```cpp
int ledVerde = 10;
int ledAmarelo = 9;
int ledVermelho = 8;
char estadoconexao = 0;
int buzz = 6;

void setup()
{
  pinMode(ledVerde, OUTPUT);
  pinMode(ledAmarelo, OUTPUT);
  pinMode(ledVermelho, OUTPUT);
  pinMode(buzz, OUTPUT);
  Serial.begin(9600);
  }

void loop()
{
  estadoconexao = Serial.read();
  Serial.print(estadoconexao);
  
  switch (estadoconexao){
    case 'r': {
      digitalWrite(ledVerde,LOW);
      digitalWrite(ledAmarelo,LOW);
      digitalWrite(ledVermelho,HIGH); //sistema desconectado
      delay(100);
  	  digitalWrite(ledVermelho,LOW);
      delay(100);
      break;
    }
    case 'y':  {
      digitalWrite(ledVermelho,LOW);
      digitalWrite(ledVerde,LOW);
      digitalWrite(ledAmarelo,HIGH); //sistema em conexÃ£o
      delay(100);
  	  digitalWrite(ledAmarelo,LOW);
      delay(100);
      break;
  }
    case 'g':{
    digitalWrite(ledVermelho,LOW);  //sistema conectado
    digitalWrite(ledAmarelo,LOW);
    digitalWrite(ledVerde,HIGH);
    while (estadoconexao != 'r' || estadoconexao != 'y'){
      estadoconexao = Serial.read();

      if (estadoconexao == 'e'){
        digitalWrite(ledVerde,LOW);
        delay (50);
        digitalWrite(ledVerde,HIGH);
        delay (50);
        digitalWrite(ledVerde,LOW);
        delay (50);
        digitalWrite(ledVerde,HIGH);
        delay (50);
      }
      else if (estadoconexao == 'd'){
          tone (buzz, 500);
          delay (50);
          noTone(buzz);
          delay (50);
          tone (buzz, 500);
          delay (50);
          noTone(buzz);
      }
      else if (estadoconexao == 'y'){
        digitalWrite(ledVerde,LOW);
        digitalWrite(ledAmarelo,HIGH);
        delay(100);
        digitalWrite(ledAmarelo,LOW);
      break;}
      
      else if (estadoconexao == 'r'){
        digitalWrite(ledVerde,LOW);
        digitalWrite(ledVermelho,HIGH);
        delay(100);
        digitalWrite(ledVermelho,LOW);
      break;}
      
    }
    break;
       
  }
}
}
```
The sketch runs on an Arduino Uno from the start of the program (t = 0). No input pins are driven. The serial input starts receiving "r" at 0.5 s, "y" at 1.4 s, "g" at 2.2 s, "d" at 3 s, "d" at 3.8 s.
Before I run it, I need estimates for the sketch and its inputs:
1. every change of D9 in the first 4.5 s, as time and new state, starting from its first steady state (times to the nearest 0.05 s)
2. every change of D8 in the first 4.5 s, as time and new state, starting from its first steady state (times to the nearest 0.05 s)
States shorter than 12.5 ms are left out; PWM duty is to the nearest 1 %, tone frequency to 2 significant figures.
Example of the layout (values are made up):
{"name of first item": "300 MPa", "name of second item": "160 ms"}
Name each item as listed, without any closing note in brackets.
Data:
{"every change of D9 in the first 4.5 s, as time and new state, starting from its first steady state": "0 s low; 1.4 s high; 1.5 s low", "every change of D8 in the first 4.5 s, as time and new state, starting from its first steady state": "0 s low; 0.5 s high; 0.6 s low"}
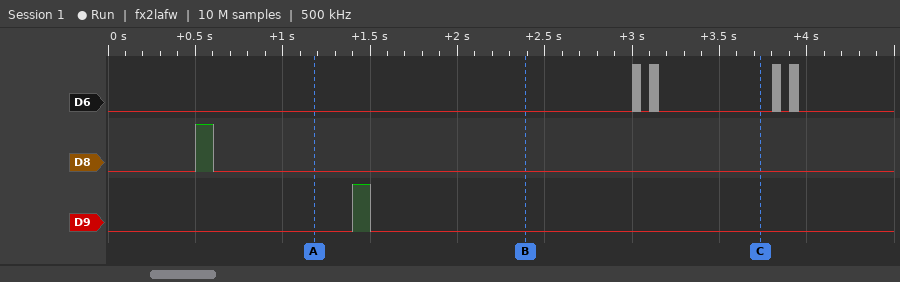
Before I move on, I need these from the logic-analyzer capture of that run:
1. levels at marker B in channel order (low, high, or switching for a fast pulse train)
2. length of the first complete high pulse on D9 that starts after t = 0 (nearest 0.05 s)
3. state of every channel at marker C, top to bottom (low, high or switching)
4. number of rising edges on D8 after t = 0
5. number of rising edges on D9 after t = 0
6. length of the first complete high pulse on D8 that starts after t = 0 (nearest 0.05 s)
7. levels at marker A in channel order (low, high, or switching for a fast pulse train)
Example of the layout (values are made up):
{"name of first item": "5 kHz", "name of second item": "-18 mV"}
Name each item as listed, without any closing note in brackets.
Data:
{"levels at marker B in channel order": "D6 low, D8 low, D9 low", "length of the first complete high pulse on D9 that starts after t = 0": "0.10 s", "state of every channel at marker C, top to bottom": "D6 low, D8 low, D9 low", "number of rising edges on D8 after t = 0": "1", "number of rising edges on D9 after t = 0": "1", "length of the first complete high pulse on D8 that starts after t = 0": "0.10 s", "levels at marker A in channel order": "D6 low, D8 low, D9 low"}
